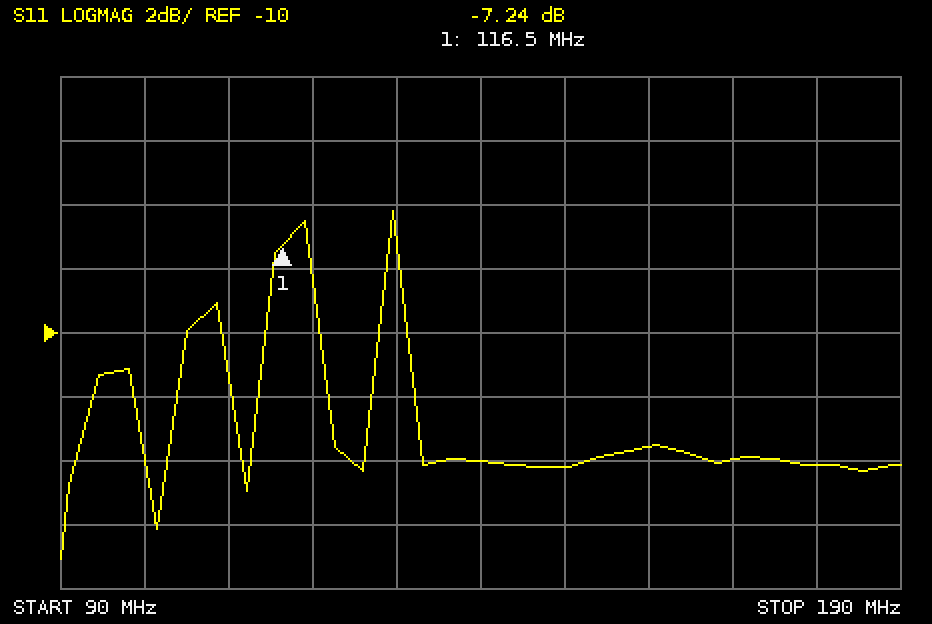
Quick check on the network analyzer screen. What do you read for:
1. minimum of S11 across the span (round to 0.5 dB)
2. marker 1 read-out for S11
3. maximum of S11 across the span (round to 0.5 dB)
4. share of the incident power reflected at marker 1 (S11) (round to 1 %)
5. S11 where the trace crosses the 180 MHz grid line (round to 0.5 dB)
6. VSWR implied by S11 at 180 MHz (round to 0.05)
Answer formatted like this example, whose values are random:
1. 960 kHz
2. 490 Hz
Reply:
1. -17.0 dB
2. -7.24 dB
3. -6.0 dB
4. 19 %
5. -14.0 dB
6. 1.50
